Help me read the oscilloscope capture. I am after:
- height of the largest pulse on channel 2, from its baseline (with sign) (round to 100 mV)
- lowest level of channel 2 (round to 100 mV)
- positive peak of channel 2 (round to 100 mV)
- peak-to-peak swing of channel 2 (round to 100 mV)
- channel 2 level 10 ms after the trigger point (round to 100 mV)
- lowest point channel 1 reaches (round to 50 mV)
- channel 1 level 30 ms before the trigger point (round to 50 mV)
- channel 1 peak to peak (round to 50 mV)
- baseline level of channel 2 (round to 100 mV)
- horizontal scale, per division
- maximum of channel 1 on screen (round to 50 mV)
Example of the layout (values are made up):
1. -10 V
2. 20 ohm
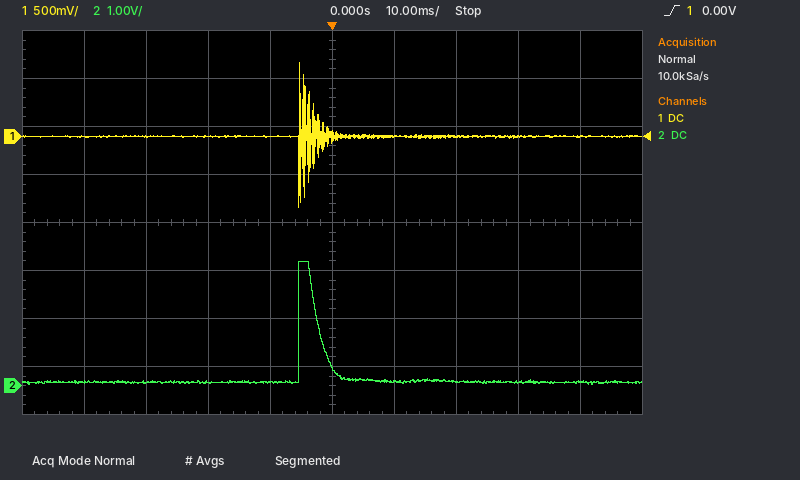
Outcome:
1. +2.5 V
2. 0.0 V
3. 2.6 V
4. 2.6 V
5. 100 mV
6. -750 mV
7. 0 mV
8. 1.50 V
9. 100 mV
10. 10 ms
11. 750 mV
